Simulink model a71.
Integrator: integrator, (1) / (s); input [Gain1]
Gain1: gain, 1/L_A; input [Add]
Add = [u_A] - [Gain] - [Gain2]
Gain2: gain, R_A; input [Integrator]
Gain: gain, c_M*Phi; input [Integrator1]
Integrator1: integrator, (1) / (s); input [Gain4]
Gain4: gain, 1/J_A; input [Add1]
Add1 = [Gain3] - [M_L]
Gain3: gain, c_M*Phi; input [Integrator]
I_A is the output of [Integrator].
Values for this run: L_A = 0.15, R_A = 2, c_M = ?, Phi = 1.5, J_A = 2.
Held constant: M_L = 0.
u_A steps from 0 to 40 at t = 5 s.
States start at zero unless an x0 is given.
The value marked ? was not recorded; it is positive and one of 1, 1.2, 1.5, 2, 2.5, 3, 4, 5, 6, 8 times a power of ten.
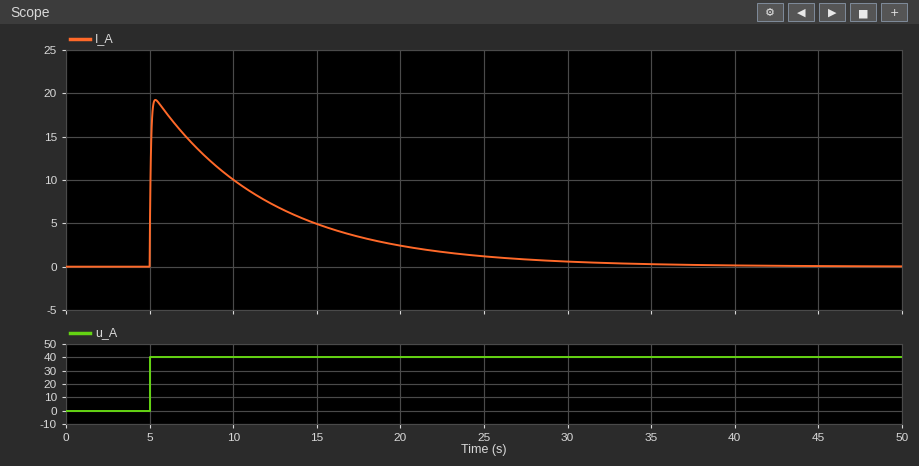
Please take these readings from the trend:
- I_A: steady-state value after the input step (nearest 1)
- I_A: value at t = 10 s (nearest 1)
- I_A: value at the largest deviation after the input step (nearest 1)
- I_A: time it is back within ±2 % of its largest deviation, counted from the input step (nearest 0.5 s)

0
10
19
28.0 s
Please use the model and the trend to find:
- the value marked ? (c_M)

0.5
